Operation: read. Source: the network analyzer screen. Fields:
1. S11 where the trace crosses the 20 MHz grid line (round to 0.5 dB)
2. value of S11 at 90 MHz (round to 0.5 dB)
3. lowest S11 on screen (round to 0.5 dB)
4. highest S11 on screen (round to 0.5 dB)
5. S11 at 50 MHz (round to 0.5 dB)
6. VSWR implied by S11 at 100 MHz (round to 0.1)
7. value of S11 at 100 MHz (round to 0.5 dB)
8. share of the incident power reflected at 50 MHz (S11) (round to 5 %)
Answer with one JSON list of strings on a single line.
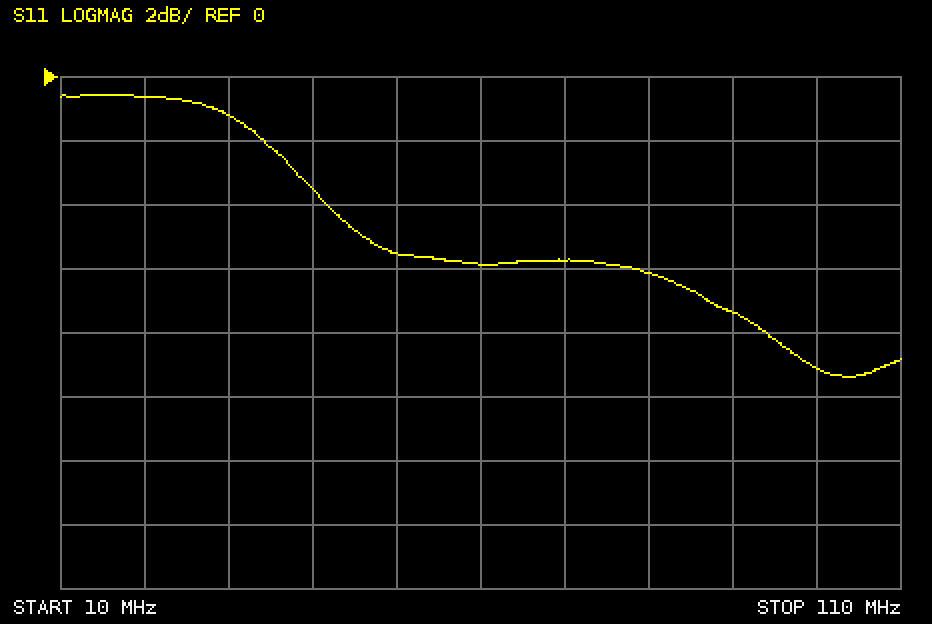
["-0.5 dB", "-7.5 dB", "-9.5 dB", "-0.5 dB", "-5.5 dB", "2.1", "-9.0 dB", "30 %"]
